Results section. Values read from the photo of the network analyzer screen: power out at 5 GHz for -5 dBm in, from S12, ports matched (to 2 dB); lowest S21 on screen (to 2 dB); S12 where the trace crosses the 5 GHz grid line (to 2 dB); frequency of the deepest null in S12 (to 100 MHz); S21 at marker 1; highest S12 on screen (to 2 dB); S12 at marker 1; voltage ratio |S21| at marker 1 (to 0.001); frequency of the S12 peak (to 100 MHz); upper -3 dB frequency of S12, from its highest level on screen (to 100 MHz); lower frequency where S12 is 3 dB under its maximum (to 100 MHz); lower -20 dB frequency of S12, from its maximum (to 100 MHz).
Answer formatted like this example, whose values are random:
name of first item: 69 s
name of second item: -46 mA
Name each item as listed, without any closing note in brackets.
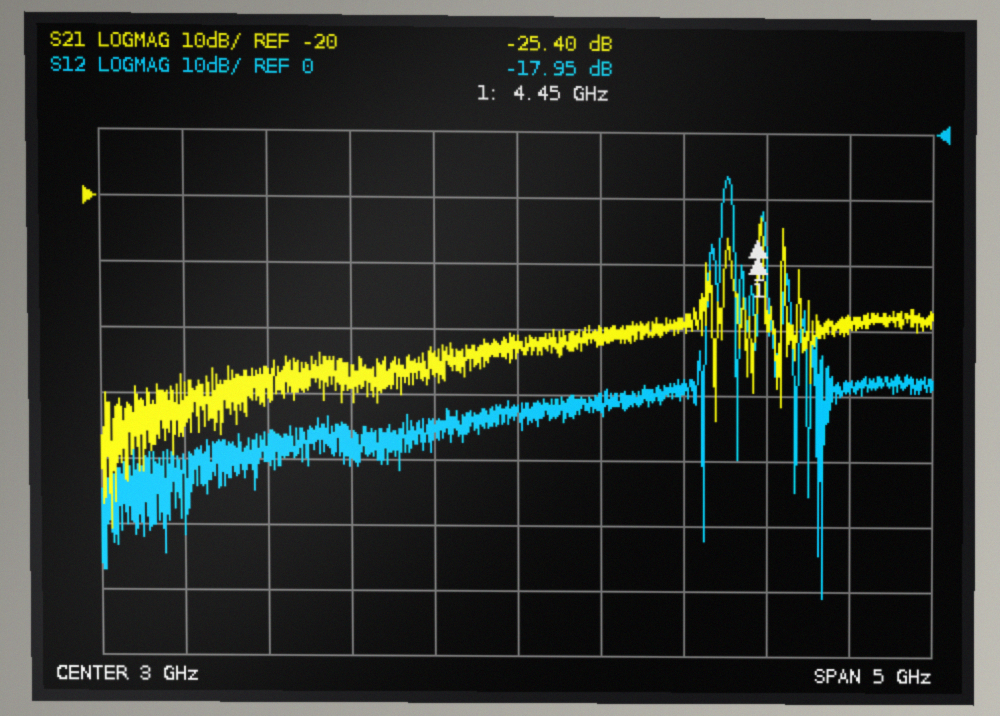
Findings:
power out at 5 GHz for -5 dBm in, from S12, ports matched: -44 dBm
lowest S21 on screen: -70 dB
S12 where the trace crosses the 5 GHz grid line: -38 dB
frequency of the deepest null in S12: 4.8 GHz
S21 at marker 1: -25.40 dB
highest S12 on screen: -6 dB
S12 at marker 1: -17.95 dB
voltage ratio |S21| at marker 1: 0.054
frequency of the S12 peak: 4.3 GHz
upper -3 dB frequency of S12, from its highest level on screen: 4.3 GHz
lower frequency where S12 is 3 dB under its maximum: 4.2 GHz
lower -20 dB frequency of S12, from its maximum: 4.1 GHz
